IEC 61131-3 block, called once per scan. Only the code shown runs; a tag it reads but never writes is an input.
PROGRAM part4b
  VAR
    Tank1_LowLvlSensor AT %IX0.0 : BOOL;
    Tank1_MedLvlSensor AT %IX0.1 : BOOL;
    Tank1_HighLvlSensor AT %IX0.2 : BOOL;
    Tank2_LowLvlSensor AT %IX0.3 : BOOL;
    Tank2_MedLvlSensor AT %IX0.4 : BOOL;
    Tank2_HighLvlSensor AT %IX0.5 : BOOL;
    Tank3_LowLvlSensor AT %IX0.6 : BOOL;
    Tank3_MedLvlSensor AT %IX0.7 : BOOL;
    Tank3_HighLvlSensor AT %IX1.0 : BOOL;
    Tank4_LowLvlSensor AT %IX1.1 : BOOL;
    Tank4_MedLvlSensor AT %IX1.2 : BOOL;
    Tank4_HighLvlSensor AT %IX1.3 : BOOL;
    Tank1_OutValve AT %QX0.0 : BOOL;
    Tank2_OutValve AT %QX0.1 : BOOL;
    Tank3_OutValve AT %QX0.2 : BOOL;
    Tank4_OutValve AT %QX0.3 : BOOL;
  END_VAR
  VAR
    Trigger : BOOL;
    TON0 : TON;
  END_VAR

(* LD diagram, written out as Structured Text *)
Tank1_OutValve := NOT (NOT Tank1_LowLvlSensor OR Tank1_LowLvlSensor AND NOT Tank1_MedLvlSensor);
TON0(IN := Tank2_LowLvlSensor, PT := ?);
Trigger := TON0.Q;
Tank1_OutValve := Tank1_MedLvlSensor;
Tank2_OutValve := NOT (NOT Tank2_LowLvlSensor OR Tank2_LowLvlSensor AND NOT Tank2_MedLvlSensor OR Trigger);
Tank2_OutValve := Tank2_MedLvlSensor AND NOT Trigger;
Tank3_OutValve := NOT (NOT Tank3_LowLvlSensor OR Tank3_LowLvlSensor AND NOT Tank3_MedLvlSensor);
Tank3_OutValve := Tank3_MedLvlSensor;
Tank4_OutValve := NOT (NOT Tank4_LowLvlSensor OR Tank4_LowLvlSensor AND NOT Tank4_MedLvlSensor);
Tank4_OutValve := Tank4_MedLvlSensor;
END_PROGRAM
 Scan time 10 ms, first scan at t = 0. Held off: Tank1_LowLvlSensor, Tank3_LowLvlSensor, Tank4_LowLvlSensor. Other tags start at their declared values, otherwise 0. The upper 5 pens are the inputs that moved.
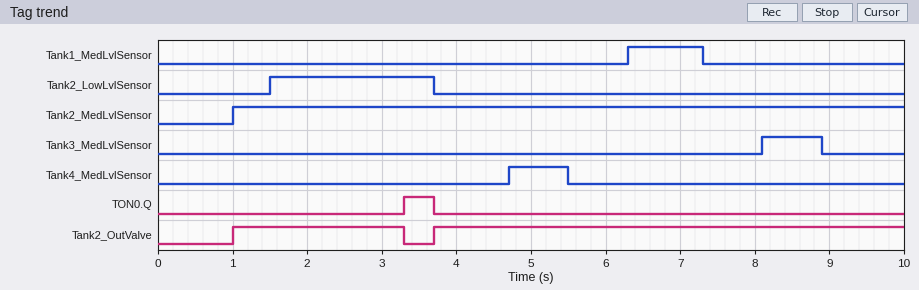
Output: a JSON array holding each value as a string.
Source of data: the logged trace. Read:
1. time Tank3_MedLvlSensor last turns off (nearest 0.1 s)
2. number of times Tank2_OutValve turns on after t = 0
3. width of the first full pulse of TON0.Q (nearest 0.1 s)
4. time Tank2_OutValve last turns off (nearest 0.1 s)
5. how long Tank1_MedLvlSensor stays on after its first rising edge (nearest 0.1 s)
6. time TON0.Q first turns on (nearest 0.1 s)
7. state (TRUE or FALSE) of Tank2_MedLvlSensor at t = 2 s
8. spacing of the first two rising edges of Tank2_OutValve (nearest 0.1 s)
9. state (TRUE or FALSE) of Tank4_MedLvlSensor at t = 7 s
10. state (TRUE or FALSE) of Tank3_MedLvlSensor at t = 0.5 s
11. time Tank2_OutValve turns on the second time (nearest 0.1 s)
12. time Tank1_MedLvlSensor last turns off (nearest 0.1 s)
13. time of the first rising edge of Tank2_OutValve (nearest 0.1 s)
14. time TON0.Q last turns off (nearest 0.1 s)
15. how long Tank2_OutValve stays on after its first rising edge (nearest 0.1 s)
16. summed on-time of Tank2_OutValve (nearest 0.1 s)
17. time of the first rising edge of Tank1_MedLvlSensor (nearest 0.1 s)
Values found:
["8.9 s", "2", "0.4 s", "3.3 s", "1.0 s", "3.3 s", "TRUE", "2.7 s", "FALSE", "FALSE", "3.7 s", "7.3 s", "1.0 s", "3.7 s", "2.3 s", "8.6 s", "6.3 s"]
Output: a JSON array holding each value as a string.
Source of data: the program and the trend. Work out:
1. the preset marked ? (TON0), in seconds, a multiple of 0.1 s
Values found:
["1.8 s"]
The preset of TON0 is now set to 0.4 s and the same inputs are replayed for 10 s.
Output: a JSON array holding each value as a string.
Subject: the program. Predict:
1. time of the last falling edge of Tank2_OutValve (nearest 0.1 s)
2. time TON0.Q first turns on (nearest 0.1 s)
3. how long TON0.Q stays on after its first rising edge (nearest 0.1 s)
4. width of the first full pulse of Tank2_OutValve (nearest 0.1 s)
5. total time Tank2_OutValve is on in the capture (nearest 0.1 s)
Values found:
["1.9 s", "1.9 s", "1.8 s", "0.9 s", "7.2 s"]
